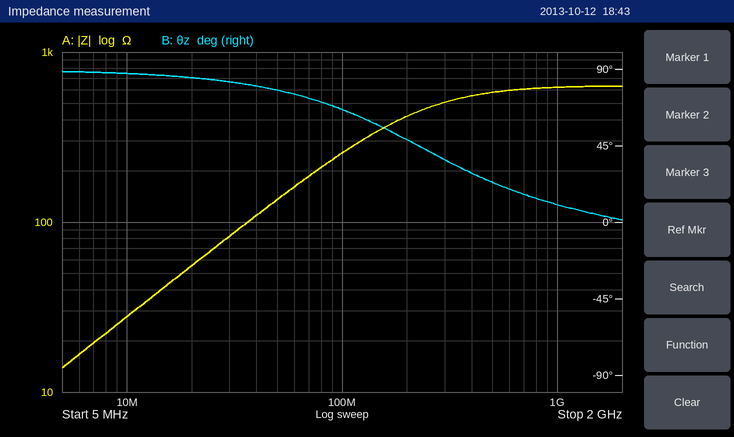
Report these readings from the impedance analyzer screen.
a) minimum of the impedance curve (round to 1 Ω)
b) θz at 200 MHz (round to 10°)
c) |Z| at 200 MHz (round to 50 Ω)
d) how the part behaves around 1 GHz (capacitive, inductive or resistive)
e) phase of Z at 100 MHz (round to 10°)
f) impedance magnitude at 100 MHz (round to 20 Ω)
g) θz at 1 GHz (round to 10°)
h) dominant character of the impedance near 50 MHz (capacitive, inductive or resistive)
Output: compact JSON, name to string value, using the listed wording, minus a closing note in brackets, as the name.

{"minimum of the impedance curve": "14 Ω", "θz at 200 MHz": "50°", "|Z| at 200 MHz": "400 Ω", "how the part behaves around 1 GHz": "resistive", "phase of Z at 100 MHz": "70°", "impedance magnitude at 100 MHz": "260 Ω", "θz at 1 GHz": "10°", "dominant character of the impedance near 50 MHz": "inductive"}
